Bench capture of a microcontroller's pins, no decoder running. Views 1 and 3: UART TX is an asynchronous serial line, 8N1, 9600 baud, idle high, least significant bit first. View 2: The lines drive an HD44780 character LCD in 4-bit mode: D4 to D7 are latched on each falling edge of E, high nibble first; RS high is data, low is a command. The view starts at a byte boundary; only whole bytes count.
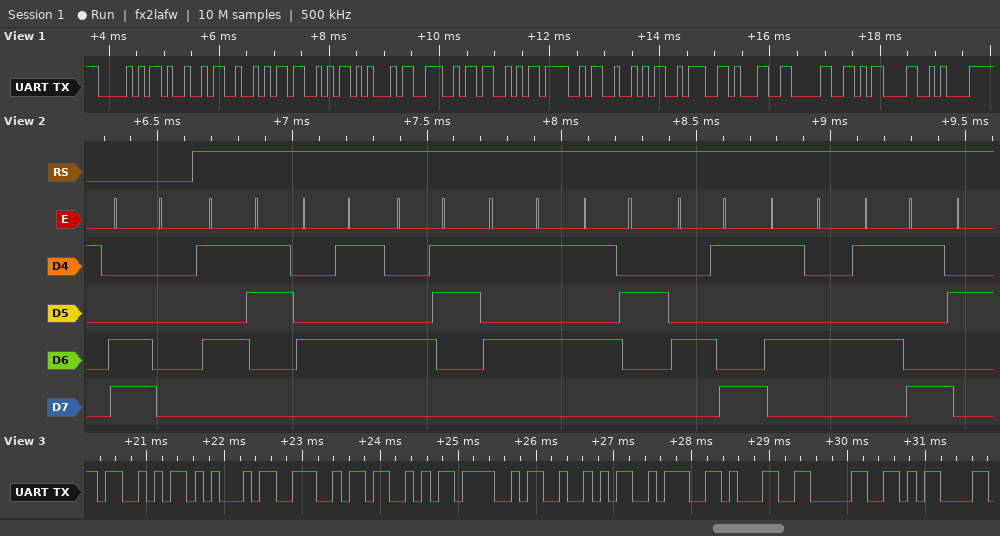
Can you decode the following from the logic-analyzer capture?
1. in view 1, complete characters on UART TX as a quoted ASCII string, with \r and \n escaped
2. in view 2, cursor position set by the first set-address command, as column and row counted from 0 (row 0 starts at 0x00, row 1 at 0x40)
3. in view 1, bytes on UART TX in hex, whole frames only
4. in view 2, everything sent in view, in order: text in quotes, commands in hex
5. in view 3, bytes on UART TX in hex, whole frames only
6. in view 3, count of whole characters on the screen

"PIRSENSOR:10\r\n"
column 0, row 1
50 49 52 53 45 4E 53 4F 52 3A 31 30 0D 0A
0xC0 "SECURITY"
53 45 4E 53 4F 52 3A 31 30 0D
10
